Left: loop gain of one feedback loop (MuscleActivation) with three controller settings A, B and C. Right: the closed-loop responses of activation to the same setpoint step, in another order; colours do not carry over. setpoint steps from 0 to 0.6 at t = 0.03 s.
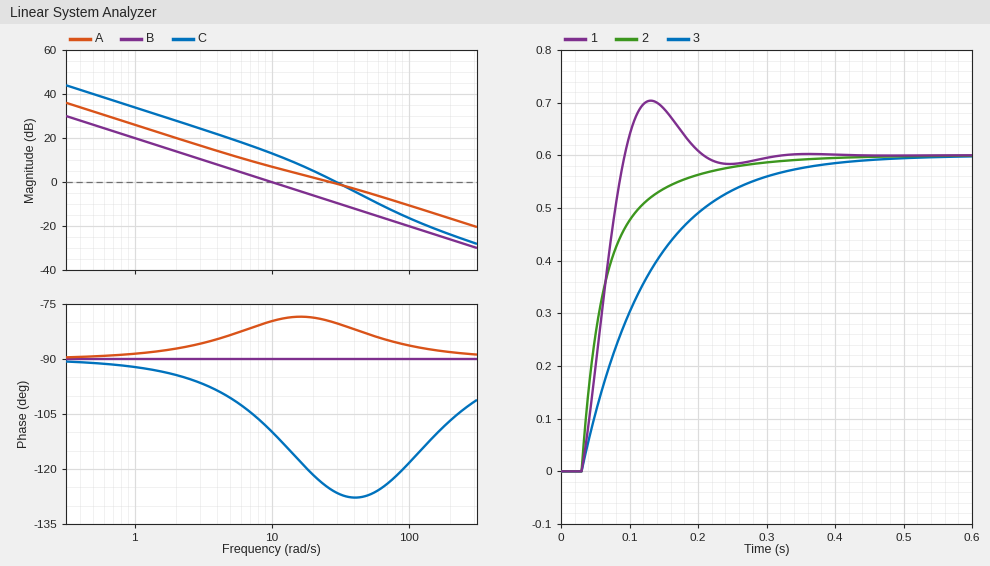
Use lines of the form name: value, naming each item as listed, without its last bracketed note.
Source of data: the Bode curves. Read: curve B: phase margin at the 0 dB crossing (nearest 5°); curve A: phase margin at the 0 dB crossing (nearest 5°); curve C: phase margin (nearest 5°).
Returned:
curve B: phase margin at the 0 dB crossing: 90°
curve A: phase margin at the 0 dB crossing: 100°
curve C: phase margin: 55°
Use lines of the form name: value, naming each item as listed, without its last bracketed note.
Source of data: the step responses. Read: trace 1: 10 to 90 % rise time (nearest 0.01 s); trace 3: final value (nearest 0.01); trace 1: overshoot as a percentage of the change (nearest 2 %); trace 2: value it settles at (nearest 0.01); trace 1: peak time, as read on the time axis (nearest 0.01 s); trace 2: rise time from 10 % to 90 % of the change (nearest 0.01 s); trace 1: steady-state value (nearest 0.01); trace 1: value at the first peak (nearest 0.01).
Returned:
trace 1: 10 to 90 % rise time: 0.05 s
trace 3: final value: 0.60
trace 1: overshoot as a percentage of the change: 18 %
trace 2: value it settles at: 0.60
trace 1: peak time, as read on the time axis: 0.13 s
trace 2: rise time from 10 % to 90 % of the change: 0.12 s
trace 1: steady-state value: 0.60
trace 1: value at the first peak: 0.70
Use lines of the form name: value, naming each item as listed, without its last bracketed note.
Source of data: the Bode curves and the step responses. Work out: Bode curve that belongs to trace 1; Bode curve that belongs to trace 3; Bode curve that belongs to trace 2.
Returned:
Bode curve that belongs to trace 1: C
Bode curve that belongs to trace 3: B
Bode curve that belongs to trace 2: A
